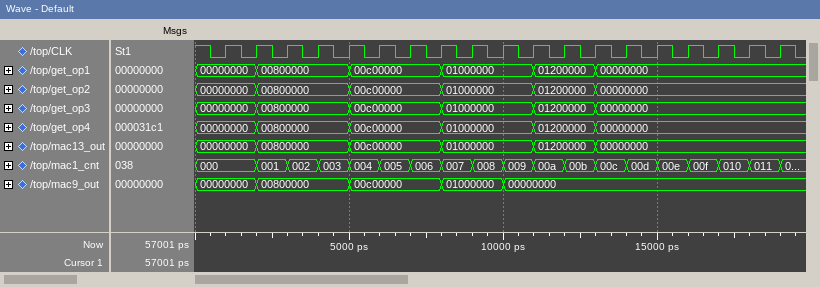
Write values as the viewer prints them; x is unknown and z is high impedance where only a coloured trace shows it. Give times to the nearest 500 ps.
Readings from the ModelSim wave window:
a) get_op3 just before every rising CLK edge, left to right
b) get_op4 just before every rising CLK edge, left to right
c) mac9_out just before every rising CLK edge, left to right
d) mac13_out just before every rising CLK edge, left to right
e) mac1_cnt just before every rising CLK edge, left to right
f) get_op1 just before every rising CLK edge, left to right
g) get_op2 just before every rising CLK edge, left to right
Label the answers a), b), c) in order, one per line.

a) 00000000, 00000000, 00800000, 00800000, 00800000, 00c00000, 00c00000, 00c00000, 01000000, 01000000, 01000000, 01200000, 01200000, 00000000, 00000000, 00000000, 00000000, 00000000, 00000000
b) 00000000, 00000000, 00800000, 00800000, 00800000, 00c00000, 00c00000, 00c00000, 01000000, 01000000, 01000000, 01200000, 01200000, 00000000, 00000000, 00000000, 00000000, 00000000, 00000000
c) 00000000, 00000000, 00800000, 00800000, 00800000, 00c00000, 00c00000, 00c00000, 01000000, 01000000, 00000000, 00000000, 00000000, 00000000, 00000000, 00000000, 00000000, 00000000, 00000000
d) 00000000, 00000000, 00800000, 00800000, 00800000, 00c00000, 00c00000, 00c00000, 01000000, 01000000, 01000000, 01200000, 01200000, 00000000, 00000000, 00000000, 00000000, 00000000, 00000000
e) 000, 000, 001, 002, 003, 004, 005, 006, 007, 008, 009, 00a, 00b, 00c, 00d, 00e, 00f, 010, 011
f) 00000000, 00000000, 00800000, 00800000, 00800000, 00c00000, 00c00000, 00c00000, 01000000, 01000000, 01000000, 01200000, 01200000, 00000000, 00000000, 00000000, 00000000, 00000000, 00000000
g) 00000000, 00000000, 00800000, 00800000, 00800000, 00c00000, 00c00000, 00c00000, 01000000, 01000000, 01000000, 01200000, 01200000, 00000000, 00000000, 00000000, 00000000, 00000000, 00000000
